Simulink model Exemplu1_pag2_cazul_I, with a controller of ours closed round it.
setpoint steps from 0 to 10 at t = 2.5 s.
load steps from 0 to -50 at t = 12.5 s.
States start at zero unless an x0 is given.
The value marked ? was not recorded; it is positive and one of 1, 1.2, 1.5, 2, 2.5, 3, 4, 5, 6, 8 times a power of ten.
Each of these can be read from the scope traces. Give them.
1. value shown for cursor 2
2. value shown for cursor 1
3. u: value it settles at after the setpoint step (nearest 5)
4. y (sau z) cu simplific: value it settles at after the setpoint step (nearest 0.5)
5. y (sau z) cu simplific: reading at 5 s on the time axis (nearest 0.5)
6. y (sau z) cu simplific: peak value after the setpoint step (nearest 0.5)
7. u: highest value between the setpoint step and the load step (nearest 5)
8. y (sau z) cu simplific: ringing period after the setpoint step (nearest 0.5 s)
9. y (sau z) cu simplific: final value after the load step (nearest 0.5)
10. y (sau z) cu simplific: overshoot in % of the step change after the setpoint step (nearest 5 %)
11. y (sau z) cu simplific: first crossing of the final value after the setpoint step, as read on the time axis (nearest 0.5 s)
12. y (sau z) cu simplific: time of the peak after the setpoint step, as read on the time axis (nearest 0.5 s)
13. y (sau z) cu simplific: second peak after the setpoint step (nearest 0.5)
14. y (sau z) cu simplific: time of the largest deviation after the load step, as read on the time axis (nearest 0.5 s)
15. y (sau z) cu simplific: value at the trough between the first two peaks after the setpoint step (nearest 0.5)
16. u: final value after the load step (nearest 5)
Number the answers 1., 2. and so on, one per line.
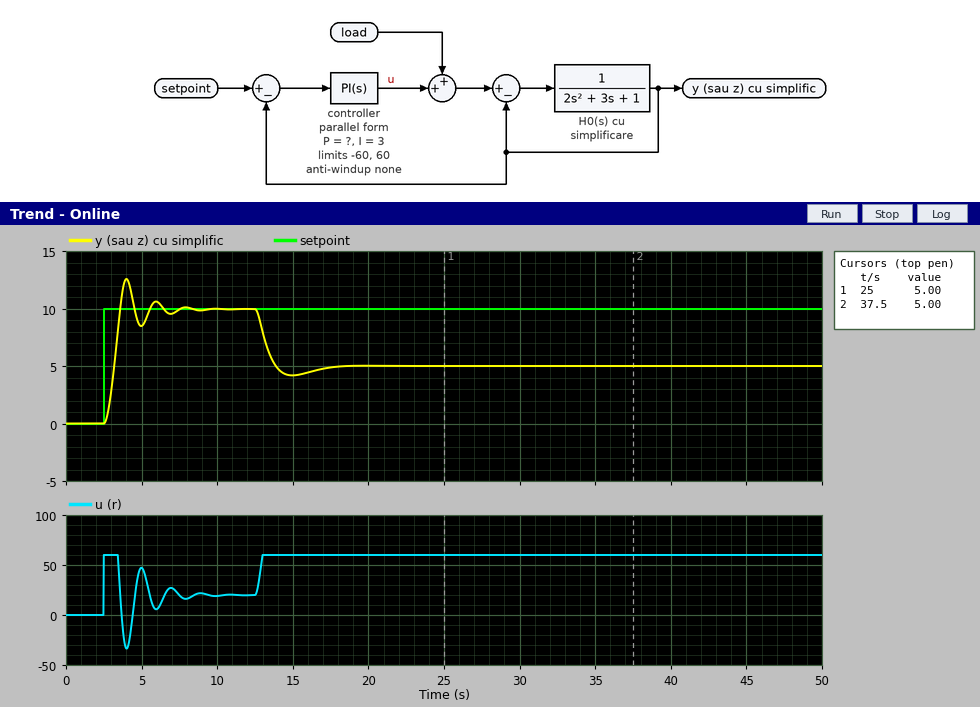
1. 5.00
2. 5.00
3. 20
4. 10.0
5. 8.5
6. 12.5
7. 60
8. 2.0 s
9. 5.0
10. 25 %
11. 3.5 s
12. 4.0 s
13. 10.5
14. 15.0 s
15. 8.5
16. 60
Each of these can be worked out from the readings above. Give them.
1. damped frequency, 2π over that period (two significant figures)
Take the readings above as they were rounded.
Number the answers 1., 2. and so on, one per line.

1. 3.1 rad/s
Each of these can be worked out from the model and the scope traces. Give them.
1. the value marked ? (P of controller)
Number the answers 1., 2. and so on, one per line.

1. 20
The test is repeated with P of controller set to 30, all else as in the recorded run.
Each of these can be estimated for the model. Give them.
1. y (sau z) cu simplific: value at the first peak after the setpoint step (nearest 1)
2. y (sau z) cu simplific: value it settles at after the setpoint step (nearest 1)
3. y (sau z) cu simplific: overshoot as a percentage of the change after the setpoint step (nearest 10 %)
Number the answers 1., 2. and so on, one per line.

1. 12
2. 10
3. 20 %
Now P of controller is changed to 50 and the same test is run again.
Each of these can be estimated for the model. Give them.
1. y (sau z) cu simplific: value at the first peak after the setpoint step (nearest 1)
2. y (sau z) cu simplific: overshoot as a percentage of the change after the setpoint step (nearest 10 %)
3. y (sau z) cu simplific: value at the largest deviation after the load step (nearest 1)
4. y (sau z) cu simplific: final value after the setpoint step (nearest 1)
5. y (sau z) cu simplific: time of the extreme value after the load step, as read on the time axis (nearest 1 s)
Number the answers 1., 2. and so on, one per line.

1. 12
2. 20 %
3. 5
4. 10
5. 16 s
